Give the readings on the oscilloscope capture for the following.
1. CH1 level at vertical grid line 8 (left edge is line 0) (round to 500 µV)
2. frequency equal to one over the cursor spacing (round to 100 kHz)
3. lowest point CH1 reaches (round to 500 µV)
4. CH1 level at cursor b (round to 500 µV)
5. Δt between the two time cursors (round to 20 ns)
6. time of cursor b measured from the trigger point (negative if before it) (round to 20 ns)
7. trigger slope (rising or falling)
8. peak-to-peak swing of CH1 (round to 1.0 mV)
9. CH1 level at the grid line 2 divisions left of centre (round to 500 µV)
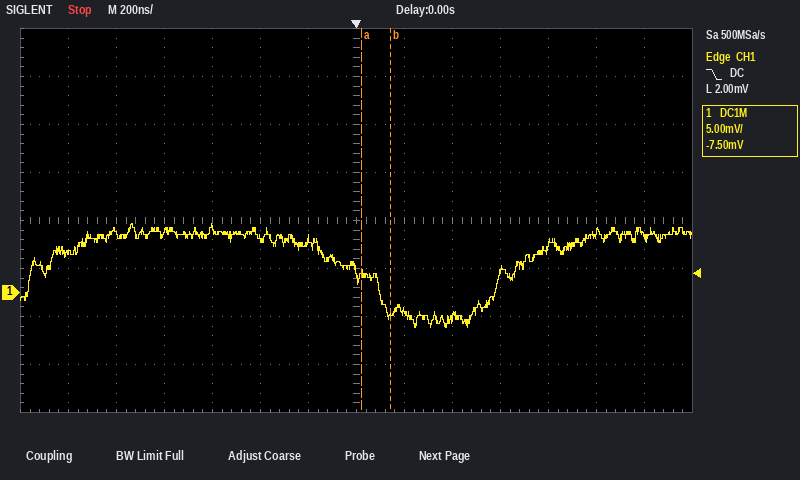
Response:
-2.0 mV
8.3 MHz
-3.5 mV
-2.5 mV
120 ns
+140 ns
falling
11.0 mV
5.5 mV
